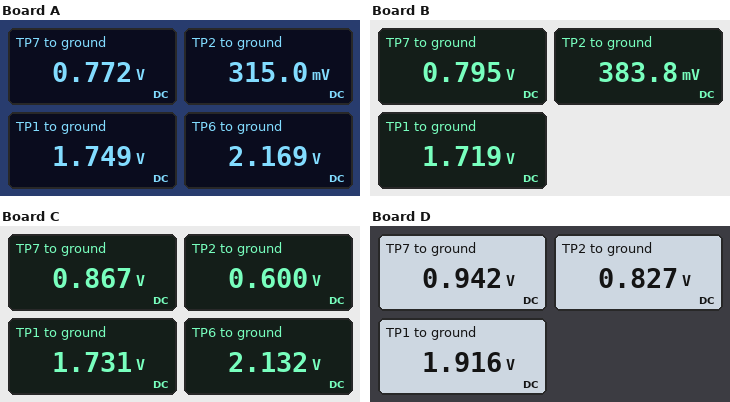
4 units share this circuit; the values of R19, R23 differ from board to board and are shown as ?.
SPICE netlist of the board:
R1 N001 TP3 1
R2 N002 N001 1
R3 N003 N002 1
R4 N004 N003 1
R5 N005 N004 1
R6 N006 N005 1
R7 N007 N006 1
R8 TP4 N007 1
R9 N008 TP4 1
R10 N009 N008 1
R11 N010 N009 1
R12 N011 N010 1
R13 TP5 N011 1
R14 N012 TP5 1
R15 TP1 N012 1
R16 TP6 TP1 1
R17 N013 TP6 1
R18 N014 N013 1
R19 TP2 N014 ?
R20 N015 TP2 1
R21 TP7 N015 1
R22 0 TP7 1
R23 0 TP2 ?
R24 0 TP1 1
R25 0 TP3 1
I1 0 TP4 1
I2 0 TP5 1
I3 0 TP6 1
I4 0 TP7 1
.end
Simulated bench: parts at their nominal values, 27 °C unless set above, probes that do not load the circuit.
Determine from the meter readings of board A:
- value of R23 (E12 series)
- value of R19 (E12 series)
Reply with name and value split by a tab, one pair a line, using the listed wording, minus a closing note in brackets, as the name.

value of R23	0.39 Ω
value of R19	1.2 Ω
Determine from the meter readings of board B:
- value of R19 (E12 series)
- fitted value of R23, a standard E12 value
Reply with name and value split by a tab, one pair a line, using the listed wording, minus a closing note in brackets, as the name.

value of R19	0.82 Ω
fitted value of R23, a standard E12 value	0.47 Ω
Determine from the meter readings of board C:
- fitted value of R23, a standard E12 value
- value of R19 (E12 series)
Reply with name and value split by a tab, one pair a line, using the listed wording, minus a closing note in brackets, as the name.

fitted value of R23, a standard E12 value	0.82 Ω
value of R19	0.56 Ω
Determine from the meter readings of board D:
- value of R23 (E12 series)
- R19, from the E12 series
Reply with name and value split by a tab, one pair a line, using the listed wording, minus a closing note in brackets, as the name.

value of R23	1.8 Ω
R19, from the E12 series	2.2 Ω
